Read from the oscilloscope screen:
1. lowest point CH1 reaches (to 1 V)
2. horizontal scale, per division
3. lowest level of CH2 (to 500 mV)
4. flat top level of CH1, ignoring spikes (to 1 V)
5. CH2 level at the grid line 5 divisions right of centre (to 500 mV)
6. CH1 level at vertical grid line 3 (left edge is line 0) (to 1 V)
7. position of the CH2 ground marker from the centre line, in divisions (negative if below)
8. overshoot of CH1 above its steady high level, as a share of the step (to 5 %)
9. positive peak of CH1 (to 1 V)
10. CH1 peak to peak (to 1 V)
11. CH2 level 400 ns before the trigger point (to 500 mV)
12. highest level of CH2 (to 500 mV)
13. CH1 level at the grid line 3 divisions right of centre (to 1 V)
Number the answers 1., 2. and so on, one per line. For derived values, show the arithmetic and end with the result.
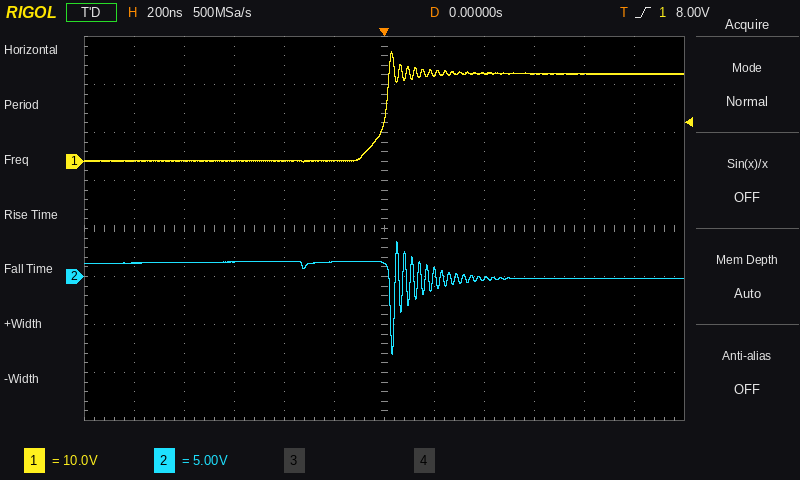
1. 0 V
2. 200 ns
3. -8.0 V
4. 18 V
5. 0.0 V
6. 0 V
7. -1.0 div
8. 25 %
9. 23 V
10. 23 V − (0 V) = 23 V
11. 1.5 V
12. 3.5 V
13. 18 V
